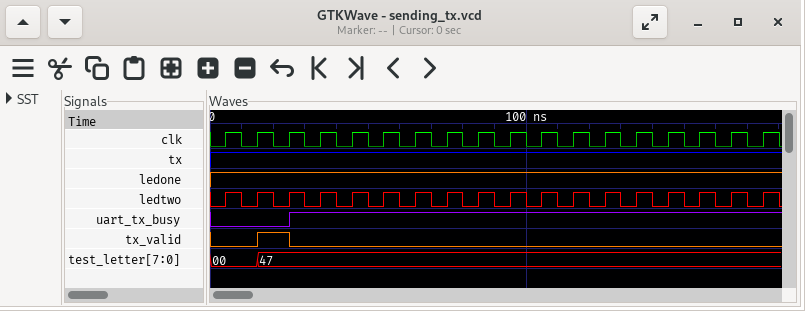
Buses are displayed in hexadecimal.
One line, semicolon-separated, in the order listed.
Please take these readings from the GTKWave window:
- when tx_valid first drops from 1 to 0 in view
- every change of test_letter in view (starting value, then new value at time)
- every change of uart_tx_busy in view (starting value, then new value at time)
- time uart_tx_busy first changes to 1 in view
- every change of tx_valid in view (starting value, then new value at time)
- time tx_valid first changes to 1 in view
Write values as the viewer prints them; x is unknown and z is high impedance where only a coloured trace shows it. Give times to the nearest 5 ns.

25 ns; 00, 47 at 15 ns; 0, 1 at 25 ns; 25 ns; 0, 1 at 15 ns, 0 at 25 ns; 15 ns
